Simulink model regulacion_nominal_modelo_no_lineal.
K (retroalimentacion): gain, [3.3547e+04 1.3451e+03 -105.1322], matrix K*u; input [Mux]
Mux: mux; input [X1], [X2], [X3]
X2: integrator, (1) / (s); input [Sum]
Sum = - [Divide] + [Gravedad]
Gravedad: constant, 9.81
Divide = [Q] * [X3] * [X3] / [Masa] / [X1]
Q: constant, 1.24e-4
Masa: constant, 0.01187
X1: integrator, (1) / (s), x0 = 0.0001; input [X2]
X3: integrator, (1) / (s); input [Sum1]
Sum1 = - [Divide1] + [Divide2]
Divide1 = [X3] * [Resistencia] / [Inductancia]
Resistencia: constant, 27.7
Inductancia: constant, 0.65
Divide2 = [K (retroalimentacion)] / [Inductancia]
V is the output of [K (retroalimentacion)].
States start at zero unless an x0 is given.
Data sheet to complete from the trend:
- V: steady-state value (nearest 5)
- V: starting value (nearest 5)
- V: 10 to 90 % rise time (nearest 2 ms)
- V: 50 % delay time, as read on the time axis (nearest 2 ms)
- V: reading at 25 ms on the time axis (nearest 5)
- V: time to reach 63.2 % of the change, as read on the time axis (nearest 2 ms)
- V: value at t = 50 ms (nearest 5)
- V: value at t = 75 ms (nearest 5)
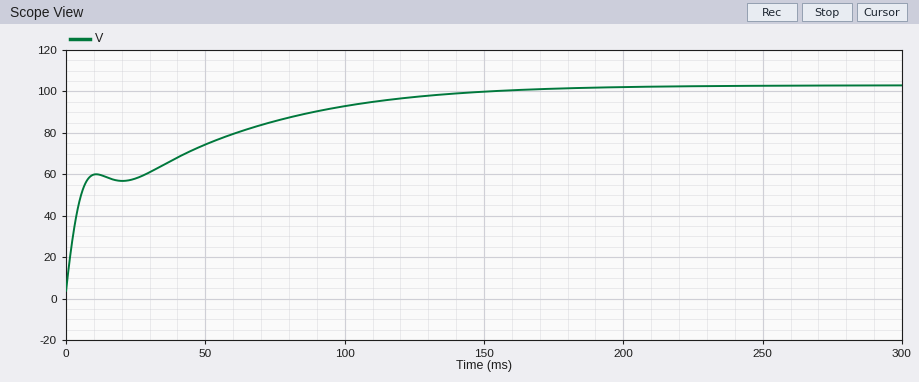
105
5
100 ms
6 ms
60
38 ms
75
85
